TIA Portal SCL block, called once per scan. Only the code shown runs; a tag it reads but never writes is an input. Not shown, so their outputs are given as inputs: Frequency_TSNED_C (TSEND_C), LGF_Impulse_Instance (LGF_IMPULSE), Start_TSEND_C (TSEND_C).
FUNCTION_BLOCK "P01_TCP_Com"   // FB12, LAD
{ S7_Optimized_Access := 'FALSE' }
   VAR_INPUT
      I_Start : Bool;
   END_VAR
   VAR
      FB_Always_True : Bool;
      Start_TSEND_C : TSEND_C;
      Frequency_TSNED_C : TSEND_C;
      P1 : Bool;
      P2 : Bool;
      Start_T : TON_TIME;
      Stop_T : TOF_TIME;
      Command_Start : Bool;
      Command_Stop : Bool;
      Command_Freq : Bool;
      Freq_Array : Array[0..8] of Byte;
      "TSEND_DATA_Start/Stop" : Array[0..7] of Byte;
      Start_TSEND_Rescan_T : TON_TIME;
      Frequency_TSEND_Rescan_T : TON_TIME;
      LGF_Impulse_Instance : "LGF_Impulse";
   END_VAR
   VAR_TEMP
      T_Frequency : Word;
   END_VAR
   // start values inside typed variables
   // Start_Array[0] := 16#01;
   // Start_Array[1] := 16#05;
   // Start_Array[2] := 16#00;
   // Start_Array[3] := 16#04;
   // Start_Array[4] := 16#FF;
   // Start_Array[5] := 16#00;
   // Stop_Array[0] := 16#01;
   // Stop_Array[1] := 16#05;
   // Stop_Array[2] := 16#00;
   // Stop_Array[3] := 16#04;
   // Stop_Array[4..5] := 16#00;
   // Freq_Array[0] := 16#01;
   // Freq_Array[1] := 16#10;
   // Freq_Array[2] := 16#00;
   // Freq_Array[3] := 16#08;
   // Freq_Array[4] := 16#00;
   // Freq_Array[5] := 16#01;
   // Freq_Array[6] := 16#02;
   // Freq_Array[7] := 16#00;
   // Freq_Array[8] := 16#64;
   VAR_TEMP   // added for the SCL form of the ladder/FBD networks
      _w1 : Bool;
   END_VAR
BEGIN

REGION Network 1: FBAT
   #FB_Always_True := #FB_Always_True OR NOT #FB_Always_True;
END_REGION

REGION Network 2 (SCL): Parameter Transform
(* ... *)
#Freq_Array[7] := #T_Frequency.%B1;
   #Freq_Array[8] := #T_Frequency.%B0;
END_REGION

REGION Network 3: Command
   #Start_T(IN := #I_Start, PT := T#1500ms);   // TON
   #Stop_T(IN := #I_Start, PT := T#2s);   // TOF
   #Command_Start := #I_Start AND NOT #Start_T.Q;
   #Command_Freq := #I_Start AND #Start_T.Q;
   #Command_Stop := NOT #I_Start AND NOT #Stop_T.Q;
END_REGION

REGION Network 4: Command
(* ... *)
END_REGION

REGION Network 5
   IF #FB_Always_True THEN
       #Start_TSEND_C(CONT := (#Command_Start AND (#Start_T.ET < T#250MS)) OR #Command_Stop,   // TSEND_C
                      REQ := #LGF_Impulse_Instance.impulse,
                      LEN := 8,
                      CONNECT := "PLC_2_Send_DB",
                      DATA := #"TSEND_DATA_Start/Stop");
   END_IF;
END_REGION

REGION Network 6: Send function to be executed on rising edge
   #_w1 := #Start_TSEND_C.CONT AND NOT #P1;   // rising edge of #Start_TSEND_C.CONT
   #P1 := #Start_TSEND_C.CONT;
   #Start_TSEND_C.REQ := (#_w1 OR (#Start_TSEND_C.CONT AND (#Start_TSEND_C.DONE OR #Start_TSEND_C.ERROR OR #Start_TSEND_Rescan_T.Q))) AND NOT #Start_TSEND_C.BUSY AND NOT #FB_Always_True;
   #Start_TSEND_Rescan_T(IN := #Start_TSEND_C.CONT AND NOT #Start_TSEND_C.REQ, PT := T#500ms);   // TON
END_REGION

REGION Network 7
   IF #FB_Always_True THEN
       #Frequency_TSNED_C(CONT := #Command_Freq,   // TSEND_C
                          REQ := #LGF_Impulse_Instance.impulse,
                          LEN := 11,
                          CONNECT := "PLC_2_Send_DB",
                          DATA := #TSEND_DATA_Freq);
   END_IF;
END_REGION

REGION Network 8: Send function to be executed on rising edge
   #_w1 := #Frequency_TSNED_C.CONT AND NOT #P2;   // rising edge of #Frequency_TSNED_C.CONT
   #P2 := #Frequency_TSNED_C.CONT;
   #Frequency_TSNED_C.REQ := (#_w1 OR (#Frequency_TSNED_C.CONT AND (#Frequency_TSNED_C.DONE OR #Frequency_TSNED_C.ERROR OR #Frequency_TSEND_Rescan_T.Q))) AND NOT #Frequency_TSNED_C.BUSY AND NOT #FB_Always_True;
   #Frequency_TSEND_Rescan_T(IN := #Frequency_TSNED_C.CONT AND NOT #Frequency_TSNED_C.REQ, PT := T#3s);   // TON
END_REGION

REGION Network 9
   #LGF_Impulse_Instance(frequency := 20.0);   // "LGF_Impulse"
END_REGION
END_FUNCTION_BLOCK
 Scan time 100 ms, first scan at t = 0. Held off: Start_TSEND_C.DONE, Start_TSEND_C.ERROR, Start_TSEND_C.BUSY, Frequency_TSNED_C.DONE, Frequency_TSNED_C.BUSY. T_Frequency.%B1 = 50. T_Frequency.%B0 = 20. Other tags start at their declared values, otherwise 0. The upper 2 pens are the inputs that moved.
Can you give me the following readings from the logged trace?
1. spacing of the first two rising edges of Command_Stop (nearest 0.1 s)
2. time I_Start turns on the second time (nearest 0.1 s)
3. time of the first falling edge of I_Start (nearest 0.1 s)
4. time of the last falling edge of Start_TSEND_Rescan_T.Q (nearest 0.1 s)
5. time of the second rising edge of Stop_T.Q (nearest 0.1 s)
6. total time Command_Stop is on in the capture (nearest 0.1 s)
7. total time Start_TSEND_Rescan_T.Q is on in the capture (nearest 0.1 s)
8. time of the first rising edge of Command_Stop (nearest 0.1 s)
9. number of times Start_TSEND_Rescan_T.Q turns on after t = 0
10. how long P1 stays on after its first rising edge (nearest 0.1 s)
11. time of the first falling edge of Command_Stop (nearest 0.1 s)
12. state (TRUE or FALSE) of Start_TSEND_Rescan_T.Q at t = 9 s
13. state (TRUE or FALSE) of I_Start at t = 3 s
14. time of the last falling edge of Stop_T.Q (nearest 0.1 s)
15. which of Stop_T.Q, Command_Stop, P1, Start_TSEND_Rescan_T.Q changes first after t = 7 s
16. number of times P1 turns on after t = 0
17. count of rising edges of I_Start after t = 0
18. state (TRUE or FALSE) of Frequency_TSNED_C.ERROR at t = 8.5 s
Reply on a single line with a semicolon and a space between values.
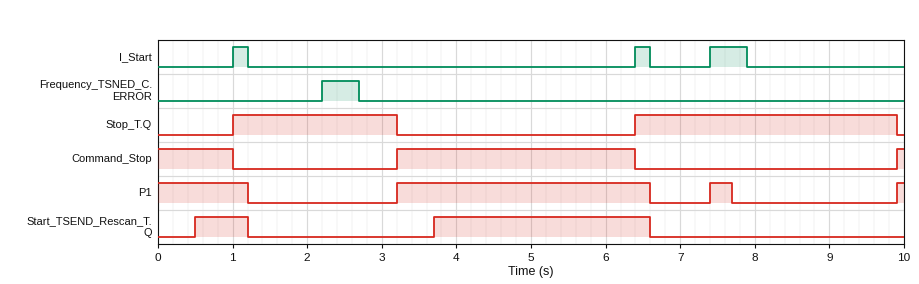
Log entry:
6.7 s; 6.4 s; 1.2 s; 6.6 s; 6.4 s; 4.3 s; 3.6 s; 3.2 s; 2; 3.4 s; 1.0 s; FALSE; FALSE; 9.9 s; P1; 3; 3; FALSE
